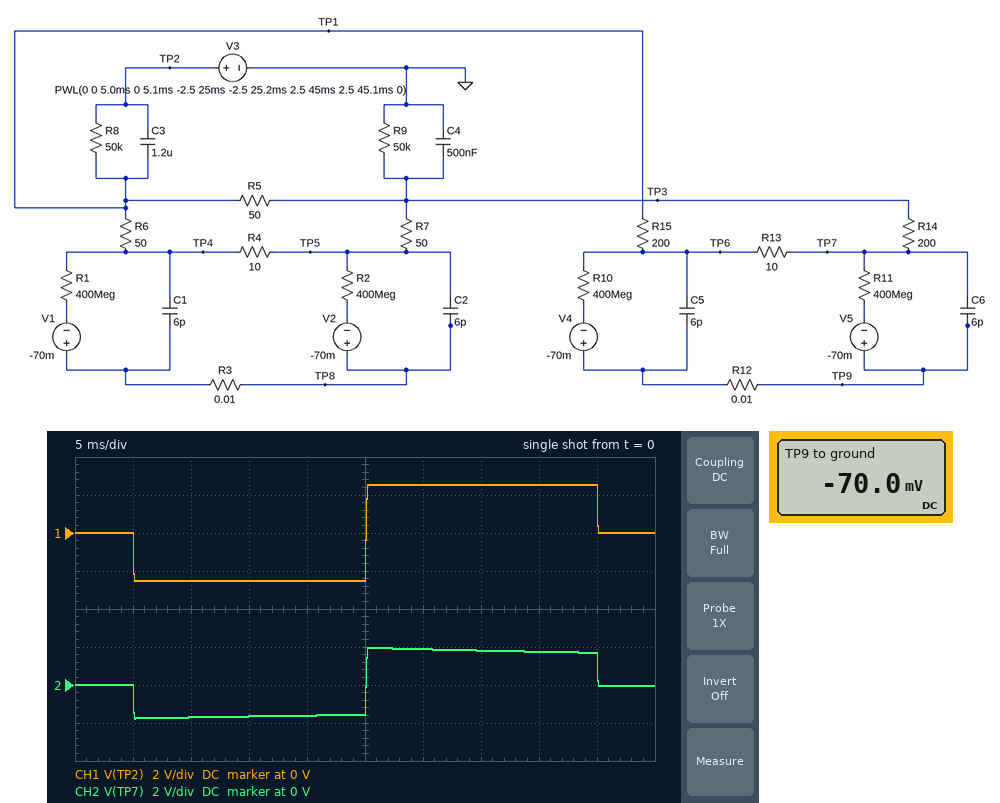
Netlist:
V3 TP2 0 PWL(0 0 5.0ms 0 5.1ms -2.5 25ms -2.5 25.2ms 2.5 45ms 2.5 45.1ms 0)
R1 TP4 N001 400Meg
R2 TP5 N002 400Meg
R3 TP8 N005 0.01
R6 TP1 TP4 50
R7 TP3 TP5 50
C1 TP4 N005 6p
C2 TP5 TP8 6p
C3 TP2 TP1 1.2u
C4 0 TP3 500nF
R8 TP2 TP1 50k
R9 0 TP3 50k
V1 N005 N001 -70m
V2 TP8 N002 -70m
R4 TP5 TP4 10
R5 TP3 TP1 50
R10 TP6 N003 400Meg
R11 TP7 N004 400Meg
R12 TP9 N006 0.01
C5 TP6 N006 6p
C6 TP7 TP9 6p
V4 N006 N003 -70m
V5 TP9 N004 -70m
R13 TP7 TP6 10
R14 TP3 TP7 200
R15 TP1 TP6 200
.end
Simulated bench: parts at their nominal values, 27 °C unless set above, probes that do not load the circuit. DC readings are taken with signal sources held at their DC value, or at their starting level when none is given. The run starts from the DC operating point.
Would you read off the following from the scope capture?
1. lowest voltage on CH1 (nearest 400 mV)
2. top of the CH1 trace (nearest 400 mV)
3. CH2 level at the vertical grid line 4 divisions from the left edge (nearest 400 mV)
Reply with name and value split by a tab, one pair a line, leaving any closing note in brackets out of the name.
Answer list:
lowest voltage on CH1	-2.4 V
top of the CH1 trace	2.4 V
CH2 level at the vertical grid line 4 divisions from the left edge	-1.6 V
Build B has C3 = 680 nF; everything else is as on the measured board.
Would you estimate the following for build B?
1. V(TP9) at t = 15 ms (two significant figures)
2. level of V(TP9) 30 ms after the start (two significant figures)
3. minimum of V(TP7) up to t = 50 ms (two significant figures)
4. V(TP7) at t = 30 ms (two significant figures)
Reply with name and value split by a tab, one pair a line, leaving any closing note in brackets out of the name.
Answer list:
V(TP9) at t = 15 ms	-1.5 V
level of V(TP9) 30 ms after the start	1.4 V
minimum of V(TP7) up to t = 50 ms	-1.4 V
V(TP7) at t = 30 ms	1.5 V
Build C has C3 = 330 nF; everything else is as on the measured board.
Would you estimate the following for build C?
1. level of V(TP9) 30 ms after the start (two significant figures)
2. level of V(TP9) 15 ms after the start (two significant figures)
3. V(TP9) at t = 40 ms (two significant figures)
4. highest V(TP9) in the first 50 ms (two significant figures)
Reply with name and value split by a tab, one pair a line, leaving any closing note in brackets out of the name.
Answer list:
level of V(TP9) 30 ms after the start	850 mV
level of V(TP9) 15 ms after the start	-1.2 V
V(TP9) at t = 40 ms	980 mV
highest V(TP9) in the first 50 ms	1.0 V
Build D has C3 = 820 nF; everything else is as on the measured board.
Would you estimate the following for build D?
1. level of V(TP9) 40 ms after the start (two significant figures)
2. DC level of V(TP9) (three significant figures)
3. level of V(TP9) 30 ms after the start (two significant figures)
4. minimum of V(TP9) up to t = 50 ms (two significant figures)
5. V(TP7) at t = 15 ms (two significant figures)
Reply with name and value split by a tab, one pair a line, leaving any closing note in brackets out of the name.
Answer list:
level of V(TP9) 40 ms after the start	1.5 V
DC level of V(TP9)	-70.0 mV
level of V(TP9) 30 ms after the start	1.6 V
minimum of V(TP9) up to t = 50 ms	-1.6 V
V(TP7) at t = 15 ms	-1.5 V
